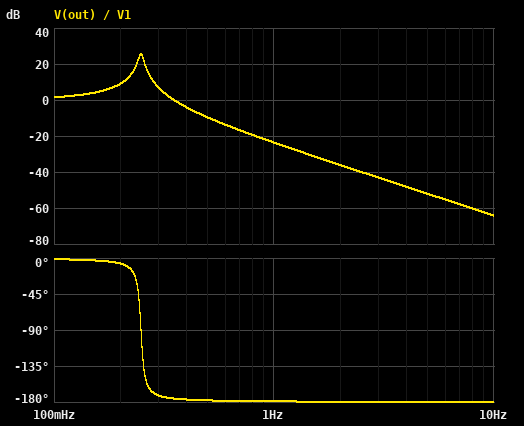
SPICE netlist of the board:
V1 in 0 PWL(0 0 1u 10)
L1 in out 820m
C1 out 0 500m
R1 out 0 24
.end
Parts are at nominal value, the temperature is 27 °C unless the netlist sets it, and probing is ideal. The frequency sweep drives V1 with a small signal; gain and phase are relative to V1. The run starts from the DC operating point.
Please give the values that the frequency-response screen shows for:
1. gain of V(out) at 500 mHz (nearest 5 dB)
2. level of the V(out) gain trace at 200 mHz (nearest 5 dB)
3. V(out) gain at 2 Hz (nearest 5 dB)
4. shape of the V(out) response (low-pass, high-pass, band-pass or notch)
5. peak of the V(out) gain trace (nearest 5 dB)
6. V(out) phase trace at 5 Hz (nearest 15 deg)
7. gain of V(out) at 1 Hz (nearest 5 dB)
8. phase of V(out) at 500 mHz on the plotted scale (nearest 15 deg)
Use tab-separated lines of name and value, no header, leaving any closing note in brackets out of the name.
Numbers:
gain of V(out) at 500 mHz	-10 dB
level of the V(out) gain trace at 200 mHz	10 dB
V(out) gain at 2 Hz	-35 dB
shape of the V(out) response	band-pass
peak of the V(out) gain trace	25 dB
V(out) phase trace at 5 Hz	-180 deg
gain of V(out) at 1 Hz	-25 dB
phase of V(out) at 500 mHz on the plotted scale	-180 deg
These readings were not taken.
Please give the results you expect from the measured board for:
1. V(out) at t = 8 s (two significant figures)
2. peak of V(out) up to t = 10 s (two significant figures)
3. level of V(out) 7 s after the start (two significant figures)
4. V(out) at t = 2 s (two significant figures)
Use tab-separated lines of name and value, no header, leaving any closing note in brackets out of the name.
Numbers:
V(out) at t = 8 s	2.9 V
peak of V(out) up to t = 10 s	19 V
level of V(out) 7 s after the start	11 V
V(out) at t = 2 s	19 V
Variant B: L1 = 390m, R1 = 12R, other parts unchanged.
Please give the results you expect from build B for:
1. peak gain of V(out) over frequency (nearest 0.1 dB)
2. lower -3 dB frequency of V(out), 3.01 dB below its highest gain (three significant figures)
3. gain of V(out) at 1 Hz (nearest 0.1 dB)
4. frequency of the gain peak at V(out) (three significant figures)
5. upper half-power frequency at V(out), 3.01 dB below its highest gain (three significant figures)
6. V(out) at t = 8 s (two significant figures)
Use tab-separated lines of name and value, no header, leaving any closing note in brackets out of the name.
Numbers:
peak gain of V(out) over frequency	22.7 dB
lower -3 dB frequency of V(out), 3.01 dB below its highest gain	346 mHz
gain of V(out) at 1 Hz	-16.5 dB
frequency of the gain peak at V(out)	360 mHz
upper half-power frequency at V(out), 3.01 dB below its highest gain	373 mHz
V(out) at t = 8 s	6.4 V
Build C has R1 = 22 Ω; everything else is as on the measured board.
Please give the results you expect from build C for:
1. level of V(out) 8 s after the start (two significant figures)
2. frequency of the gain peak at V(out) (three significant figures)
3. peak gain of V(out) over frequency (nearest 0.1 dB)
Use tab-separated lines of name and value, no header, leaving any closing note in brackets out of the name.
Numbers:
level of V(out) 8 s after the start	3.1 V
frequency of the gain peak at V(out)	248 mHz
peak gain of V(out) over frequency	24.7 dB
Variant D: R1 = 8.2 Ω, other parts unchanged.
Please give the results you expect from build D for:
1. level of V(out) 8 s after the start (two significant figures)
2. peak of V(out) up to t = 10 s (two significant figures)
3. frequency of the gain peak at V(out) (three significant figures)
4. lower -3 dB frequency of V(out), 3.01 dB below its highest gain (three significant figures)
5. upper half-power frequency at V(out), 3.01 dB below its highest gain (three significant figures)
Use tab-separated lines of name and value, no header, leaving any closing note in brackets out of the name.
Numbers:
level of V(out) 8 s after the start	6.3 V
peak of V(out) up to t = 10 s	18 V
frequency of the gain peak at V(out)	247 mHz
lower -3 dB frequency of V(out), 3.01 dB below its highest gain	227 mHz
upper half-power frequency at V(out), 3.01 dB below its highest gain	266 mHz
